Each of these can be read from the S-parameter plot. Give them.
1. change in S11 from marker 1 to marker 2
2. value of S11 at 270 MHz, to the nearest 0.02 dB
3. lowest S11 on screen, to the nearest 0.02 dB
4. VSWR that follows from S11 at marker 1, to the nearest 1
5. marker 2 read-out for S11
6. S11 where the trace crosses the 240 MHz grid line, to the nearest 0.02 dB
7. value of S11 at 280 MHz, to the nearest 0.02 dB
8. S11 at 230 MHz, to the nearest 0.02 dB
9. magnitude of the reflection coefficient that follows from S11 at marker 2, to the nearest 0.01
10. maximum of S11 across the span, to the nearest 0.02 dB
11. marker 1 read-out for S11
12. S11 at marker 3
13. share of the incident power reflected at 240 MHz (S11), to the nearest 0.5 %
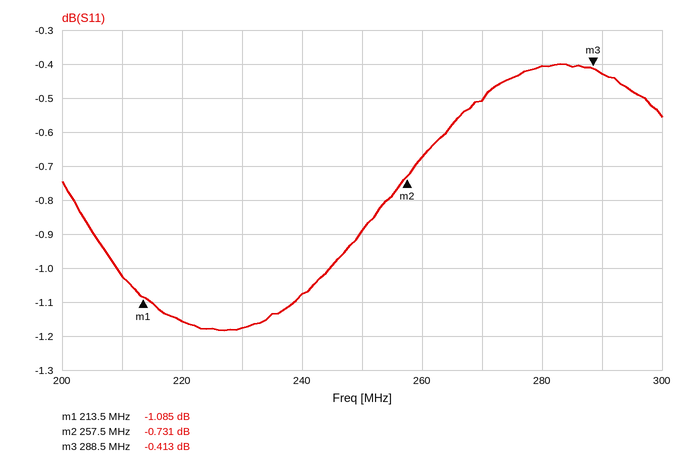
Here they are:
0.354 dB
-0.50 dB
-1.18 dB
16
-0.731 dB
-1.08 dB
-0.40 dB
-1.18 dB
0.92
-0.40 dB
-1.085 dB
-0.413 dB
78.0 %
